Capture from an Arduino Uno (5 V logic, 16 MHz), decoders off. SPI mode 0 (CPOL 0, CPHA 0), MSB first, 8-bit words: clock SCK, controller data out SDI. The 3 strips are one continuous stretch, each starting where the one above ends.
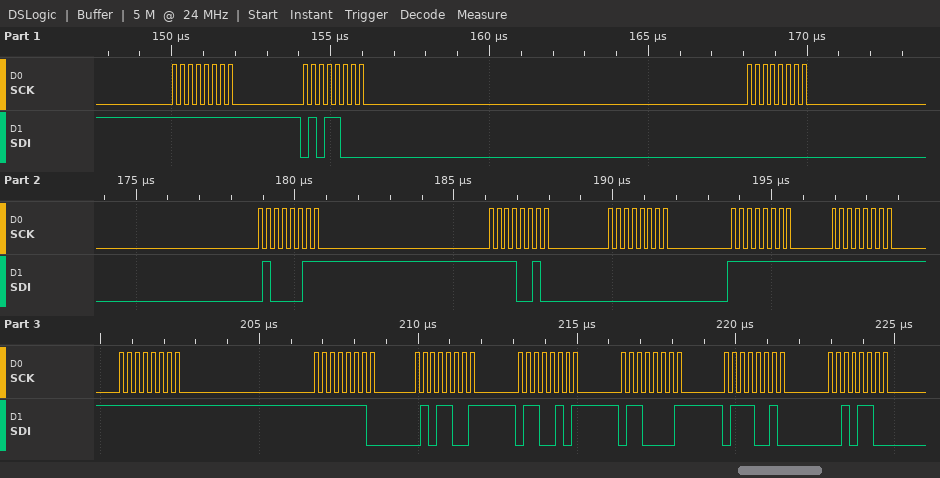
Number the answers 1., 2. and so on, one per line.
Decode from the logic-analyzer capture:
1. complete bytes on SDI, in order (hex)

1. 0xFF 0x58 0x00 0x43 0xF2 0x00 0xFF 0xFF 0xFF 0xFE 0x59 0x65 0x61 0x72 0x2C
